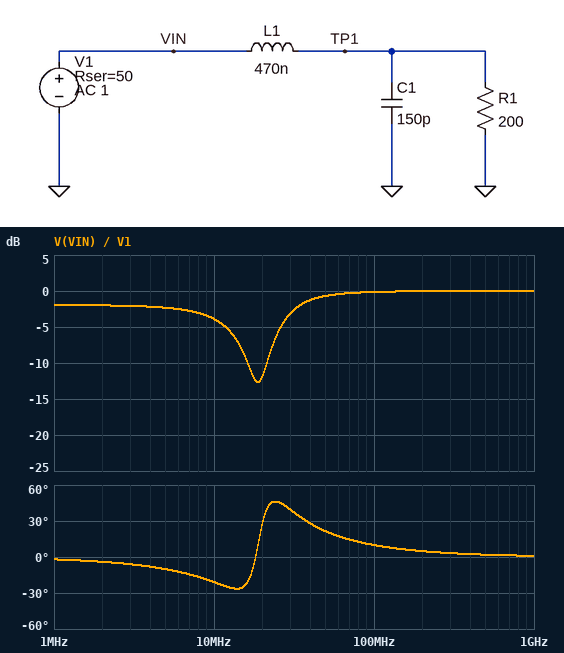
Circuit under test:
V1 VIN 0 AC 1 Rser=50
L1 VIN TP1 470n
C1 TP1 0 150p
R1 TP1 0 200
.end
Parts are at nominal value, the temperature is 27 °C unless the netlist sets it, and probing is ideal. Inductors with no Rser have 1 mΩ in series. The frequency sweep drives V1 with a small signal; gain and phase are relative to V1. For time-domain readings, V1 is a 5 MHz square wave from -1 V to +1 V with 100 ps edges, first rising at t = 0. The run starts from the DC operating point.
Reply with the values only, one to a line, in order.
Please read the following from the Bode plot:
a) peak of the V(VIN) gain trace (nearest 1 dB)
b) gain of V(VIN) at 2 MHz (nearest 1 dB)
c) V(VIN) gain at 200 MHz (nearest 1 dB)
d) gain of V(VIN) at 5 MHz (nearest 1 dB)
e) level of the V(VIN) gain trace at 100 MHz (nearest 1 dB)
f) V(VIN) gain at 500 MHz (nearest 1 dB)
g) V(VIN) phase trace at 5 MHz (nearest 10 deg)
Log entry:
0 dB
-2 dB
0 dB
-2 dB
0 dB
0 dB
-10 deg
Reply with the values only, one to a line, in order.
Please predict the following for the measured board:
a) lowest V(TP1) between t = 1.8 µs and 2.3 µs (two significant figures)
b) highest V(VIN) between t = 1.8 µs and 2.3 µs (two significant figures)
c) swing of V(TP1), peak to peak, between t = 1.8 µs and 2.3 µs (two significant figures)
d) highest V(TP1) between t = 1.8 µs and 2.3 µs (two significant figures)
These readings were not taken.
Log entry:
-1.0 V
1.2 V
2.1 V
1.0 V
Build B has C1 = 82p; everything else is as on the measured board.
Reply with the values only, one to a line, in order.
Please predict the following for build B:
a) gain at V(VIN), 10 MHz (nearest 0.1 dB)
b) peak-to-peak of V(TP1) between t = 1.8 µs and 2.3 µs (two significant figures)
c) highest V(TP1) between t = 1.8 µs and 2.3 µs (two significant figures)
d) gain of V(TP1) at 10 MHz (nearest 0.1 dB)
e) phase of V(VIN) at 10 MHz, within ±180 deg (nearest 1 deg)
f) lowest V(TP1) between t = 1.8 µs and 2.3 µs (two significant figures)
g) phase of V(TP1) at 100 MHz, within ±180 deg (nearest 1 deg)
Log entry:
-2.7 dB
2.2 V
1.1 V
-1.4 dB
-10 deg
-1.1 V
-164 deg
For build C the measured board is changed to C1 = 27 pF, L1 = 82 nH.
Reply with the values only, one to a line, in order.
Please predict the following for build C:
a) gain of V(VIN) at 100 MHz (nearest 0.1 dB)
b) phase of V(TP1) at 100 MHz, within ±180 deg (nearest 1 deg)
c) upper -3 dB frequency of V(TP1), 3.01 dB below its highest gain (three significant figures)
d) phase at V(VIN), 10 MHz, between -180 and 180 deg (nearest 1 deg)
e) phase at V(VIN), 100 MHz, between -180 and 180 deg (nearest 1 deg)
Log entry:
-12.2 dB
-71 deg
138 MHz
-4 deg
-7 deg
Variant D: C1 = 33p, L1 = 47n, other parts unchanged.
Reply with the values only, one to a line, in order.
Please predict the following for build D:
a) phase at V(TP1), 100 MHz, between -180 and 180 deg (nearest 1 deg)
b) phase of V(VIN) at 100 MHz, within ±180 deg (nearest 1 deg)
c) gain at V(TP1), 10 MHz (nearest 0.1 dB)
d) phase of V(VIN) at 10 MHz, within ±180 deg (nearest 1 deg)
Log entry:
-62 deg
-41 deg
-1.9 dB
-5 deg
